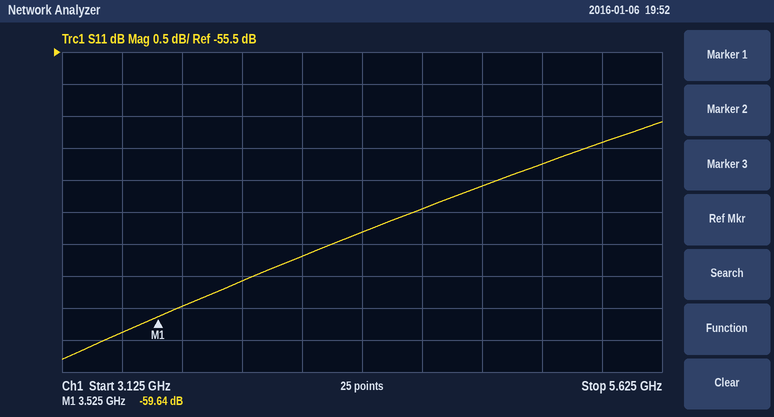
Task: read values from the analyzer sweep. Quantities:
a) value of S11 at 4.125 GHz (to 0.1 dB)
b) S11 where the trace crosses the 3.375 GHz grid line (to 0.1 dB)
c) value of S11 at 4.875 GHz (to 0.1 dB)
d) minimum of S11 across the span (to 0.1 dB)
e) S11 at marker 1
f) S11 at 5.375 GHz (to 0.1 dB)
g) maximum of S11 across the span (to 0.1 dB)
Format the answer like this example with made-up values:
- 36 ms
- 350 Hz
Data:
- -58.7 dB
- -59.9 dB
- -57.6 dB
- -60.3 dB
- -59.64 dB
- -56.9 dB
- -56.6 dB
